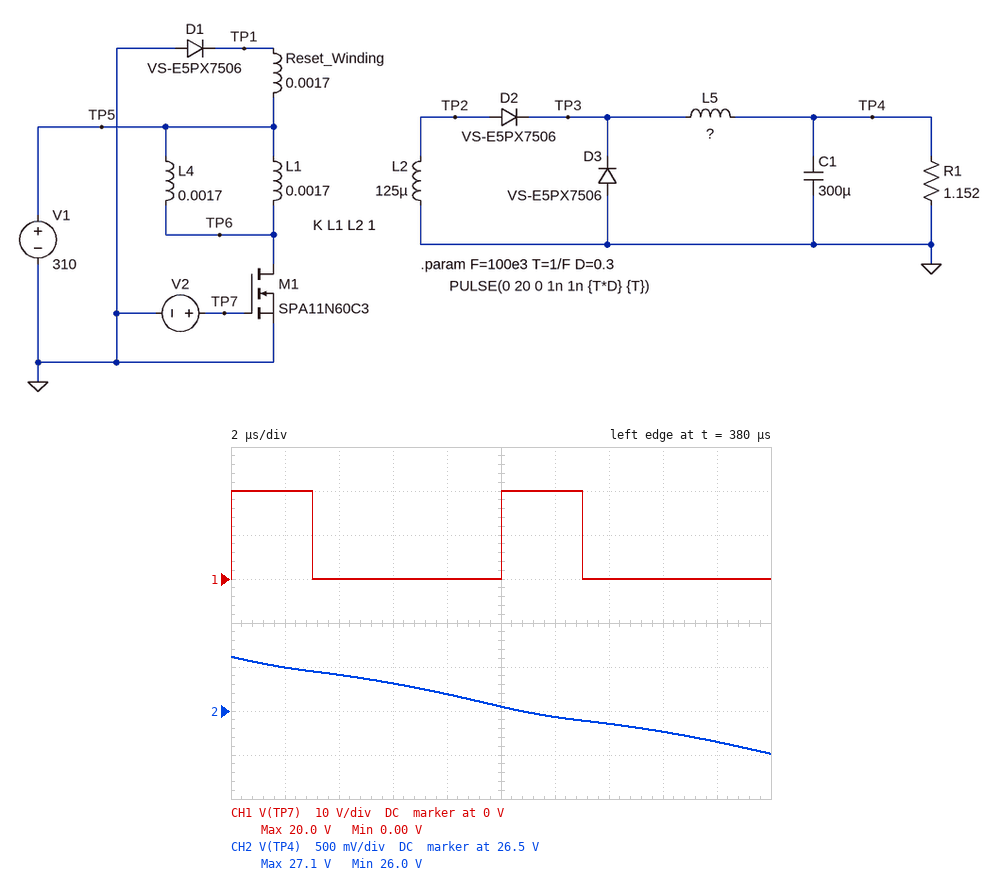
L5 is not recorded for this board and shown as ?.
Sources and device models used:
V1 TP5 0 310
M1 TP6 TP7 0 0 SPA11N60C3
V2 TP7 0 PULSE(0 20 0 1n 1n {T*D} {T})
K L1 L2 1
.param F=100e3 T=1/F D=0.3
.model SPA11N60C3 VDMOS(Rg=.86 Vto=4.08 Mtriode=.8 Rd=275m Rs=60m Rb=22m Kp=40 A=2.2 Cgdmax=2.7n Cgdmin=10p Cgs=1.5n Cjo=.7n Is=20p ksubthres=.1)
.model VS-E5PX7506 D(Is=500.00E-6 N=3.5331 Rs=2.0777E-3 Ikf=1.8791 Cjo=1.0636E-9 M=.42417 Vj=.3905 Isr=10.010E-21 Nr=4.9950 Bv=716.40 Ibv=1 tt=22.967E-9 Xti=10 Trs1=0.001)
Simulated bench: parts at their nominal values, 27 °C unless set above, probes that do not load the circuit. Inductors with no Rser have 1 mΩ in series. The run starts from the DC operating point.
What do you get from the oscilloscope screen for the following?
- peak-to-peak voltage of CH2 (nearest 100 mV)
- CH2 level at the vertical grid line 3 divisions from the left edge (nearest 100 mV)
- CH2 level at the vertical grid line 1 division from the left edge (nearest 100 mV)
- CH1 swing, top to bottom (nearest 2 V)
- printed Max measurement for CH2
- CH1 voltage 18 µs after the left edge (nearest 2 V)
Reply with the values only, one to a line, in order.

1.1 V
26.8 V
27.0 V
20 V
27.1 V
0 V
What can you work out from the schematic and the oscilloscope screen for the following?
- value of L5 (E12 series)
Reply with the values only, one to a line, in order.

15 µH
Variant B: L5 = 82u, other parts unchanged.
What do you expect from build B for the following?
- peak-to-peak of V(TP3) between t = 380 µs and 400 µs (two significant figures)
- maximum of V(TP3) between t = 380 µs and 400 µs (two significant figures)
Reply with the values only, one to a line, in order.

83 V
82 V
